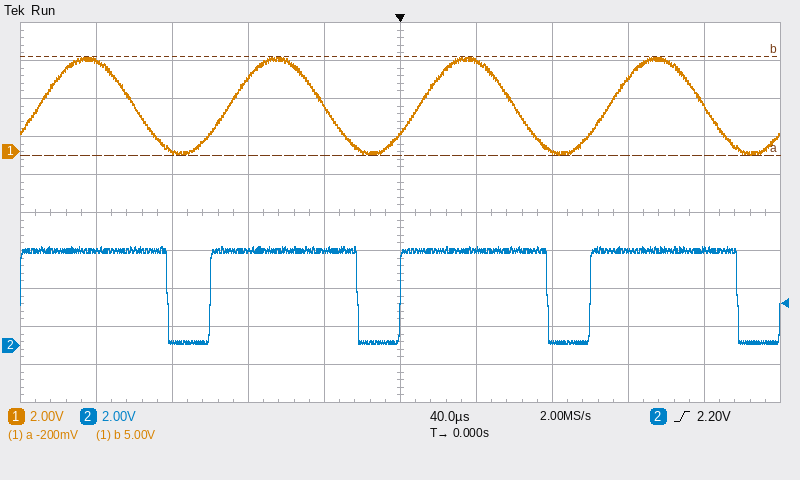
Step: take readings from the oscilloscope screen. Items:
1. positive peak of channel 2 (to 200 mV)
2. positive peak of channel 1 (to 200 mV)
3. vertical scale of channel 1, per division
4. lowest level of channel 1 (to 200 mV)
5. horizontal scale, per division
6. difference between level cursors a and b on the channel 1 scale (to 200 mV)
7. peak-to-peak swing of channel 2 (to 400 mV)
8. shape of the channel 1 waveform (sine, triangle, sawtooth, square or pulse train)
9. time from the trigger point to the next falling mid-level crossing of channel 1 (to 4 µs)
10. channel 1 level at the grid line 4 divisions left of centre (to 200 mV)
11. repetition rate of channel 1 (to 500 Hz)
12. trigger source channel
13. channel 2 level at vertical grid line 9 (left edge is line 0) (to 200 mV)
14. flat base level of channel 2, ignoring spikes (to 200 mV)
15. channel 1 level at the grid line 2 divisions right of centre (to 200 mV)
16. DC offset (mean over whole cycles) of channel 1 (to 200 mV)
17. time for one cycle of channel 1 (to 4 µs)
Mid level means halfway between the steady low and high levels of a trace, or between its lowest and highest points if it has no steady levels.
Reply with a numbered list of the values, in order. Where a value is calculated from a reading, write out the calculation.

1. 5.2 V
2. 5.0 V
3. 2 V
4. -200 mV
5. 40 µs
6. 5.2 V
7. 5.2 V
8. sine
9. 60 µs
10. 4.8 V
11. 1 / 100 µs ≈ 10.0 kHz
12. channel 2
13. 5.0 V
14. 200 mV
15. 0.0 V
16. (5.0 V + (-200 mV)) / 2 ≈ 2.4 V
17. 100 µs
